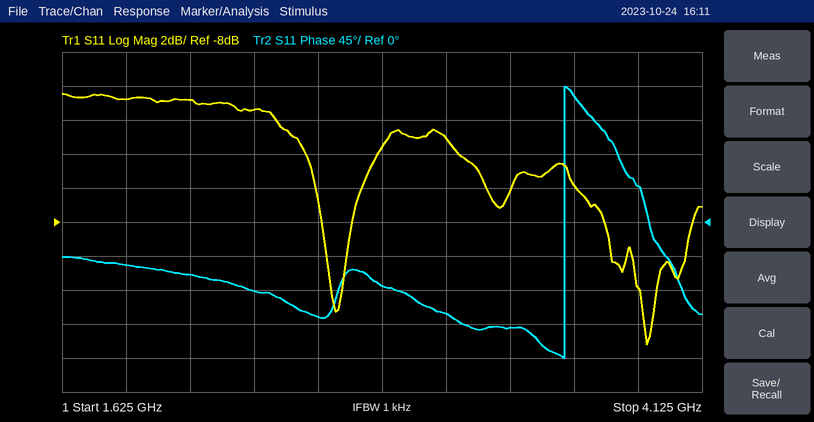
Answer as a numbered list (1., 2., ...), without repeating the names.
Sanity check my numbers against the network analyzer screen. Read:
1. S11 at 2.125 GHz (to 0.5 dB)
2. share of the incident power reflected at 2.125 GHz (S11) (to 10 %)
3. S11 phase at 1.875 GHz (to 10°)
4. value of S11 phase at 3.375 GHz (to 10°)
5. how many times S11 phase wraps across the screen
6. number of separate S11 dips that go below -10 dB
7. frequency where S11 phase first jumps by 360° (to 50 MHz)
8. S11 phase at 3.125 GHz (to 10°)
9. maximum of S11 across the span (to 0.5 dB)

1. -1.0 dB
2. 80 %
3. -60°
4. -140°
5. 1
6. 2
7. 3.60 GHz
8. -120°
9. -0.5 dB
